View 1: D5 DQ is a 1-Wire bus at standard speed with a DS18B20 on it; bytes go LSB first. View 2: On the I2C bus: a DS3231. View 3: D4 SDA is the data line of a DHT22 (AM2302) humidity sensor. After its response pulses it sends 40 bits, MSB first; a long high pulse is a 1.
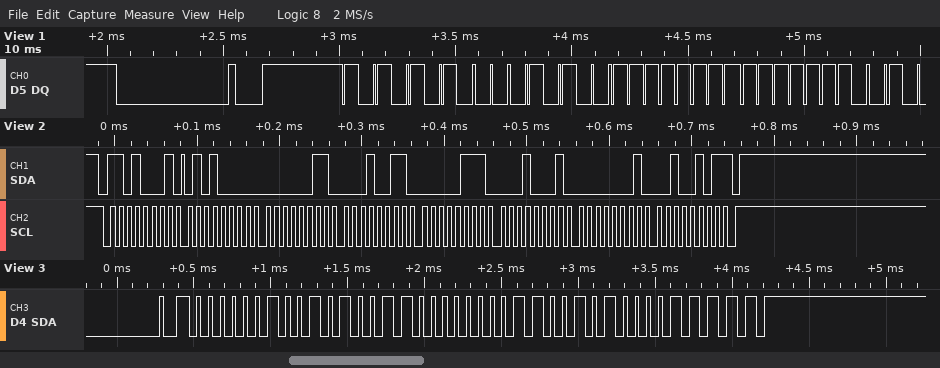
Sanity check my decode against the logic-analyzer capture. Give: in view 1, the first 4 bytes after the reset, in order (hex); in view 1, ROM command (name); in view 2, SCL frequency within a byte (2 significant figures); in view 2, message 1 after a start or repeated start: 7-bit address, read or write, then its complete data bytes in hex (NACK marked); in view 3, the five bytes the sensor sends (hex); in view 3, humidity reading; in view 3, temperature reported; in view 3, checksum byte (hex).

55 28 FF 7F
Match ROM
100 kHz
0x68 read: 50 03 13 07 11 01 25 NACK
02 53 00 CA 1F
59.5 %
20.2 °C
0x1F
